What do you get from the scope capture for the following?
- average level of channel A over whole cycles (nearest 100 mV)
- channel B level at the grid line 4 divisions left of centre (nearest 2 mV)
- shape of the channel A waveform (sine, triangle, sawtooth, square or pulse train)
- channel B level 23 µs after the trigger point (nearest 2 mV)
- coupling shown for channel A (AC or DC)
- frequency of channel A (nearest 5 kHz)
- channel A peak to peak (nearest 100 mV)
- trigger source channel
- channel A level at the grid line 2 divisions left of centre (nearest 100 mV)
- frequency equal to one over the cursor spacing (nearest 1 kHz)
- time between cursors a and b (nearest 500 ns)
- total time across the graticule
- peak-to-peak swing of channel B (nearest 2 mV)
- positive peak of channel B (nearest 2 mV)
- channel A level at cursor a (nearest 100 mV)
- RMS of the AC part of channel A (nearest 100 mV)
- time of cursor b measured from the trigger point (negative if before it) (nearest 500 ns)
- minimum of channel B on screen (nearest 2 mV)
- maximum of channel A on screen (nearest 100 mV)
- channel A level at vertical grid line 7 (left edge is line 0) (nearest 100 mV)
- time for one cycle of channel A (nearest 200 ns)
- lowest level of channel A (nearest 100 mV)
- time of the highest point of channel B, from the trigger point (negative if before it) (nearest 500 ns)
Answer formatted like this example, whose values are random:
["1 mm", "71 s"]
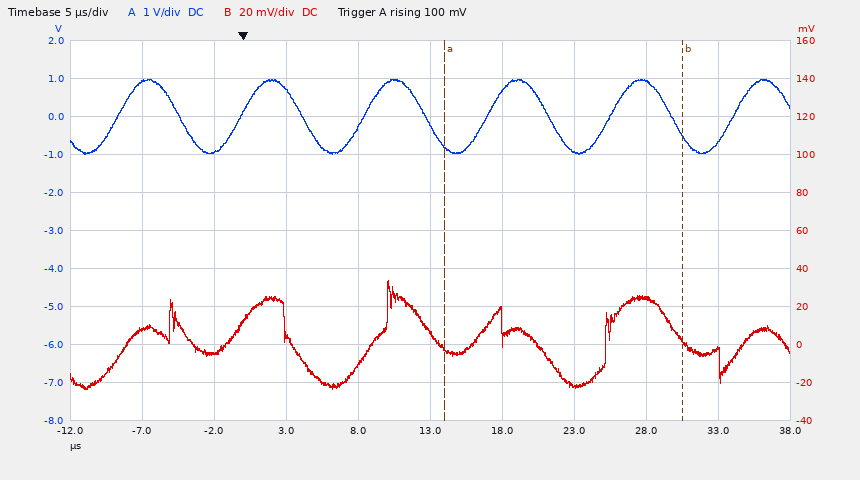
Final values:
["0.0 V", "8 mV", "sine", "-22 mV", "DC", "115 kHz", "2.0 V", "channel A", "700 mV", "61 kHz", "16.5 µs", "50 µs", "58 mV", "34 mV", "-800 mV", "700 mV", "+30.5 µs", "-24 mV", "1.0 V", "-900 mV", "8.6 µs", "-1.0 V", "+10.0 µs"]
